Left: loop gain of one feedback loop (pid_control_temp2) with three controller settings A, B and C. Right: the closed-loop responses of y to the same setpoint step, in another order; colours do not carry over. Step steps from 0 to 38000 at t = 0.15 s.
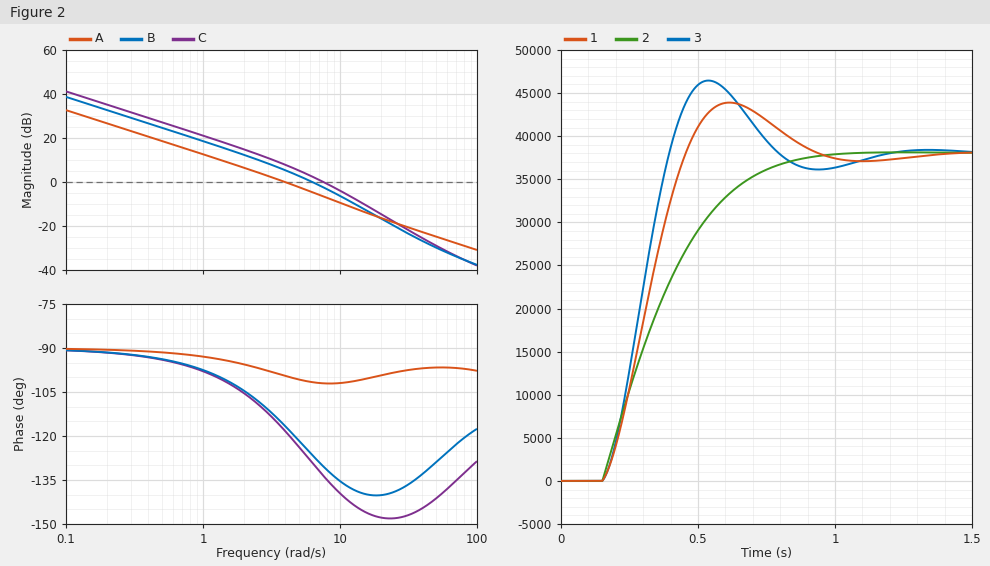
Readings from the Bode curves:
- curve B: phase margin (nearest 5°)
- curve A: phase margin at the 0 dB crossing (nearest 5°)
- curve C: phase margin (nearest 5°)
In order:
55°
80°
45°
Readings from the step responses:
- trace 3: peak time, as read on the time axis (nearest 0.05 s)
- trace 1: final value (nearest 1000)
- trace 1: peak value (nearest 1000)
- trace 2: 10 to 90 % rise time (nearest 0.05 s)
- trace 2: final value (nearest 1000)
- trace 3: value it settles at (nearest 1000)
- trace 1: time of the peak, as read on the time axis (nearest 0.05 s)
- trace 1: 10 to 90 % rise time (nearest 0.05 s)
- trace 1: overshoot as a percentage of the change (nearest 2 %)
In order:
0.55 s
38000
44000
0.45 s
38000
38000
0.60 s
0.20 s
16 %
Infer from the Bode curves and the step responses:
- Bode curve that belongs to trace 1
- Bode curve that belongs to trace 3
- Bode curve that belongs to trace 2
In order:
B
C
A
